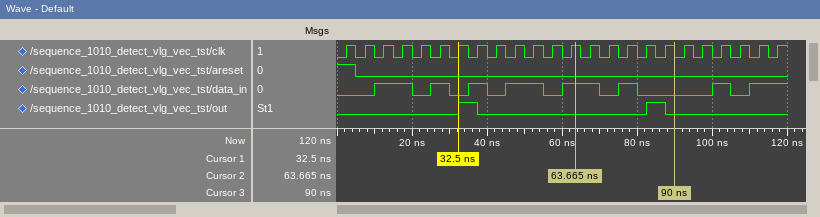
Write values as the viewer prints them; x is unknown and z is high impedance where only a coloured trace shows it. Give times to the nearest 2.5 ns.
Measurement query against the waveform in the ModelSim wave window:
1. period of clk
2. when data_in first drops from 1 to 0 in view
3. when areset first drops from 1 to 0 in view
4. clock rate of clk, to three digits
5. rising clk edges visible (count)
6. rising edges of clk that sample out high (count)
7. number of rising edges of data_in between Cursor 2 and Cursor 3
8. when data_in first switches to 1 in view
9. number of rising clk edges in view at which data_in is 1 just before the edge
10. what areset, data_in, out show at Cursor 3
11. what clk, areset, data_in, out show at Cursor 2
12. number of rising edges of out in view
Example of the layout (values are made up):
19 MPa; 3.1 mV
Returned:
5 ns; 20 ns; 5 ns; 200 MHz; 24; 2; 1; 10 ns; 12; areset=0, data_in=0, out=0; clk=1, areset=0, data_in=1, out=0; 2
